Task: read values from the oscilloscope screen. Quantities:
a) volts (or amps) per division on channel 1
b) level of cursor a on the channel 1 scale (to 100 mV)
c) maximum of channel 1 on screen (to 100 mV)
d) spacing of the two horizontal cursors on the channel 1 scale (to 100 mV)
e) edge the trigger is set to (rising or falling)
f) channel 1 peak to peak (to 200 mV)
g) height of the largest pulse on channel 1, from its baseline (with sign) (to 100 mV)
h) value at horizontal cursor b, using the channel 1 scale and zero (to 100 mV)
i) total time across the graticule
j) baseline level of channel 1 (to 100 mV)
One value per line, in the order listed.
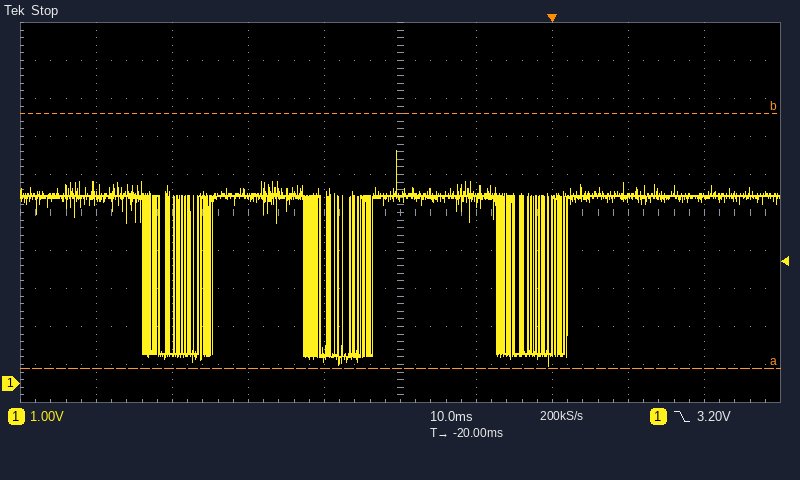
1 V
400 mV
6.1 V
6.7 V
falling
5.6 V
-4.5 V
7.1 V
100 ms
4.9 V
